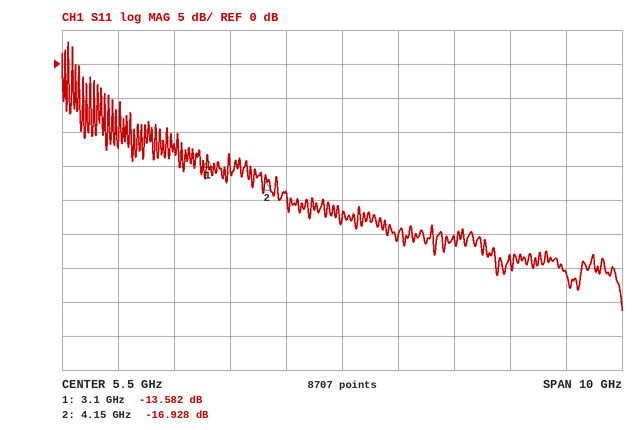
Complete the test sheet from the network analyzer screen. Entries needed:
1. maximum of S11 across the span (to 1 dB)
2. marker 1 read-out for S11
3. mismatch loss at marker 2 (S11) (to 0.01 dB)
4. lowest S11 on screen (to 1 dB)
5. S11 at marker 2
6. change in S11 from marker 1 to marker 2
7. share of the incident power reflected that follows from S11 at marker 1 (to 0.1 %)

3 dB
-13.582 dB
0.09 dB
-36 dB
-16.928 dB
-3.346 dB
4.4 %
